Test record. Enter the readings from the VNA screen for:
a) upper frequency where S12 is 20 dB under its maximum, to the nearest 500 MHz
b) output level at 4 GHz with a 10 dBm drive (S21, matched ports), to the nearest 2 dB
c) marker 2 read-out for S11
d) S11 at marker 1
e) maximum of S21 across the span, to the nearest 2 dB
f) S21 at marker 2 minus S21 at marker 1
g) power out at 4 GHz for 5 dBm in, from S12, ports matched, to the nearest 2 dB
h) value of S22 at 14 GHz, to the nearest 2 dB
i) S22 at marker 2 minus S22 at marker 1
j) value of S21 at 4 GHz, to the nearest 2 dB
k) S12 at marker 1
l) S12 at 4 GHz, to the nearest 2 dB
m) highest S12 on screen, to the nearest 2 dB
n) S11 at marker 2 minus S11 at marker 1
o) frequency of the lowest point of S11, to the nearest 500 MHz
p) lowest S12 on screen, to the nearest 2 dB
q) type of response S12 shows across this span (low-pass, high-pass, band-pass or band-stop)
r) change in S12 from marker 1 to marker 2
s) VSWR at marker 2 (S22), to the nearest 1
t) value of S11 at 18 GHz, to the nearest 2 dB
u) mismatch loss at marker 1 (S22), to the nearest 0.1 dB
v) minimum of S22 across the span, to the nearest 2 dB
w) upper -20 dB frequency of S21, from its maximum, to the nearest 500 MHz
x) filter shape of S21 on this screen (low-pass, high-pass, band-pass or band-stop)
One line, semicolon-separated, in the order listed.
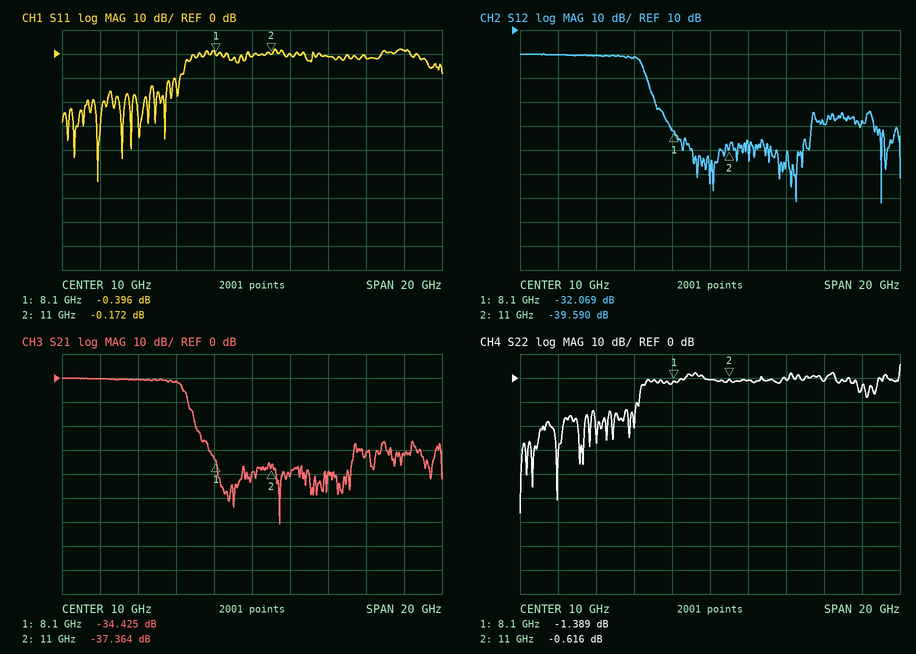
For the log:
7.0 GHz; 10 dBm; -0.172 dB; -0.396 dB; 0 dB; -2.939 dB; 4 dBm; 0 dB; 0.773 dB; 0 dB; -32.069 dB; 0 dB; 0 dB; 0.224 dB; 2.0 GHz; -62 dB; low-pass; -7.521 dB; 28; 2 dB; 5.6 dB; -56 dB; 7.0 GHz; low-pass
